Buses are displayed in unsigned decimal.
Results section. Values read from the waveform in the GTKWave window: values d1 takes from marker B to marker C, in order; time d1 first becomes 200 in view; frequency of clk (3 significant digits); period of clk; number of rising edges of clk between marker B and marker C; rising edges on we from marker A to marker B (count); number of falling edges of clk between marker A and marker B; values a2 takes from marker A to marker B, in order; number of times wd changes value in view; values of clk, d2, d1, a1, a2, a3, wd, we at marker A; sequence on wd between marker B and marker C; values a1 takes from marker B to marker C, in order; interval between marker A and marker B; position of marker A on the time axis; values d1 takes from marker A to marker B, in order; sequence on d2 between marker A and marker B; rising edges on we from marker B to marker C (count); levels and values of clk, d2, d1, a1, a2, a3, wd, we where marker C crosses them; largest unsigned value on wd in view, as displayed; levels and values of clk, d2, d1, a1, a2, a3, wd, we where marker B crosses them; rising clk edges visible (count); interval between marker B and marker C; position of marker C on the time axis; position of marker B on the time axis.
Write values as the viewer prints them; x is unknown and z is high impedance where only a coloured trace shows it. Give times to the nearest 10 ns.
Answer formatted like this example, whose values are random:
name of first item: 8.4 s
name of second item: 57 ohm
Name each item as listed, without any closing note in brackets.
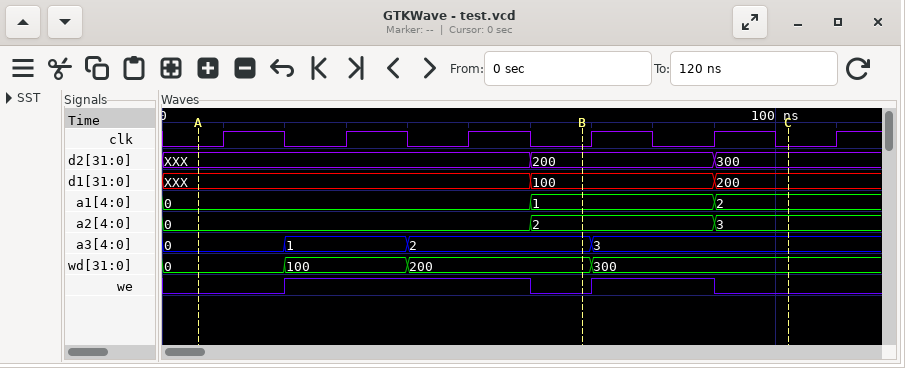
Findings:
values d1 takes from marker B to marker C, in order: 100, 200
time d1 first becomes 200 in view: 90 ns
frequency of clk: 50.0 MHz
period of clk: 20 ns
number of rising edges of clk between marker B and marker C: 2
rising edges on we from marker A to marker B: 1
number of falling edges of clk between marker A and marker B: 3
values a2 takes from marker A to marker B, in order: 0, 2
number of times wd changes value in view: 3
values of clk, d2, d1, a1, a2, a3, wd, we at marker A: clk=0, d2=XXX, d1=XXX, a1=0, a2=0, a3=0, wd=0, we=0
sequence on wd between marker B and marker C: 200, 300
values a1 takes from marker B to marker C, in order: 1, 2
interval between marker A and marker B: 60 ns
position of marker A on the time axis: 10 ns
values d1 takes from marker A to marker B, in order: XXX, 100
sequence on d2 between marker A and marker B: XXX, 200
rising edges on we from marker B to marker C: 1
levels and values of clk, d2, d1, a1, a2, a3, wd, we where marker C crosses them: clk=0, d2=300, d1=200, a1=2, a2=3, a3=3, wd=300, we=0
largest unsigned value on wd in view, as displayed: 300
levels and values of clk, d2, d1, a1, a2, a3, wd, we where marker B crosses them: clk=0, d2=200, d1=100, a1=1, a2=2, a3=2, wd=200, we=0
rising clk edges visible: 6
interval between marker B and marker C: 30 ns
position of marker C on the time axis: 100 ns
position of marker B on the time axis: 70 ns
